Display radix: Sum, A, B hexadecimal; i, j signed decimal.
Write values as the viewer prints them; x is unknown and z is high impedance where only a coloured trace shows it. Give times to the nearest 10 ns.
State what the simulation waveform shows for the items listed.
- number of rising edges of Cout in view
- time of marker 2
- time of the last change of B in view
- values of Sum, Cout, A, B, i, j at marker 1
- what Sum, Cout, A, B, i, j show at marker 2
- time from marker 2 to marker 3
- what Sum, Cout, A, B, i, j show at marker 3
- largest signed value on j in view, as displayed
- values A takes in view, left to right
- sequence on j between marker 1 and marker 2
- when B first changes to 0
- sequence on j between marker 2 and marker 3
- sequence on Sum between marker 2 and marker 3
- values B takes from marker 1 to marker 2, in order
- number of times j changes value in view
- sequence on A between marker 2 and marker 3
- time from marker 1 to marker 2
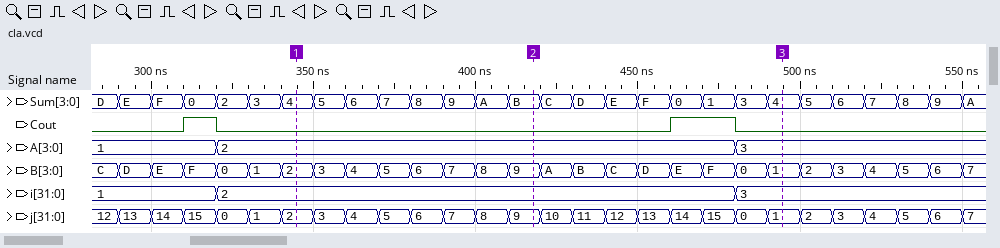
2
420 ns
550 ns
Sum=4, Cout=0, A=2, B=2, i=2, j=2
Sum=B, Cout=0, A=2, B=9, i=2, j=9
80 ns
Sum=4, Cout=0, A=3, B=1, i=3, j=1
15
1, 2, 3
2, 3, 4, 5, 6, 7, 8, 9
320 ns
9, 10, 11, 12, 13, 14, 15, 0, 1
B, C, D, E, F, 0, 1, 3, 4
2, 3, 4, 5, 6, 7, 8, 9
27
2, 3
70 ns
